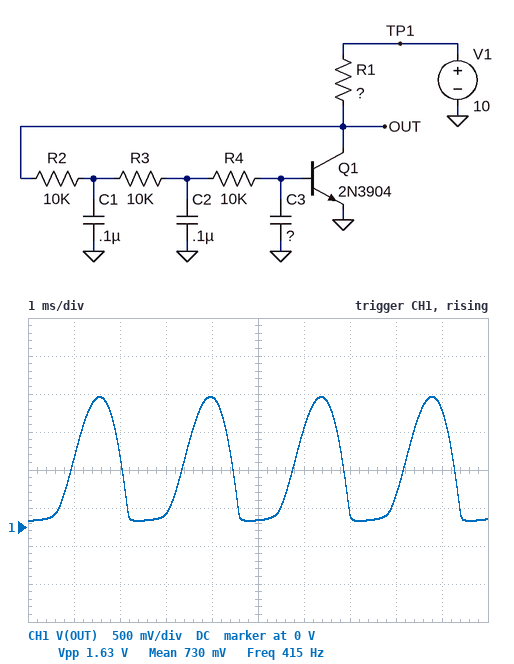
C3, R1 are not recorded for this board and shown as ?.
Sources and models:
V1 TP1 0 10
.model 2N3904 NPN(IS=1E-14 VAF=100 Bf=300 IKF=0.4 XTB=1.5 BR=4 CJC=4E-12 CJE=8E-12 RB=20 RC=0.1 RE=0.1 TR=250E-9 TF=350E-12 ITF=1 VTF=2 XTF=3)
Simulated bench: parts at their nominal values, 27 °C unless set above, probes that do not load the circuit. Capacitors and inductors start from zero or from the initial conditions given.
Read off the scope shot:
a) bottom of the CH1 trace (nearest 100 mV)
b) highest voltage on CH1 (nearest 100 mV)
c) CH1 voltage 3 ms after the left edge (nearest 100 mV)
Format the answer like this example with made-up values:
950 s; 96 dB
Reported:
100 mV; 1.7 V; 200 mV
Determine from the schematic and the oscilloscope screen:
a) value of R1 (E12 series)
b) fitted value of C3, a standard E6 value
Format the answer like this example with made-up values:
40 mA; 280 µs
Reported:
15 kΩ; 330 nF
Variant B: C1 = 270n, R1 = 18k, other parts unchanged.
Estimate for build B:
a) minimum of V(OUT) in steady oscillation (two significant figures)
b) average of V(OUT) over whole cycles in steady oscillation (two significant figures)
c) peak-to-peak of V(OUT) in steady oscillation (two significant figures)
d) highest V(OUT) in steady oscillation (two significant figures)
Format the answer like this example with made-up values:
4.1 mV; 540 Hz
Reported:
87 mV; 720 mV; 1.5 V; 1.6 V
